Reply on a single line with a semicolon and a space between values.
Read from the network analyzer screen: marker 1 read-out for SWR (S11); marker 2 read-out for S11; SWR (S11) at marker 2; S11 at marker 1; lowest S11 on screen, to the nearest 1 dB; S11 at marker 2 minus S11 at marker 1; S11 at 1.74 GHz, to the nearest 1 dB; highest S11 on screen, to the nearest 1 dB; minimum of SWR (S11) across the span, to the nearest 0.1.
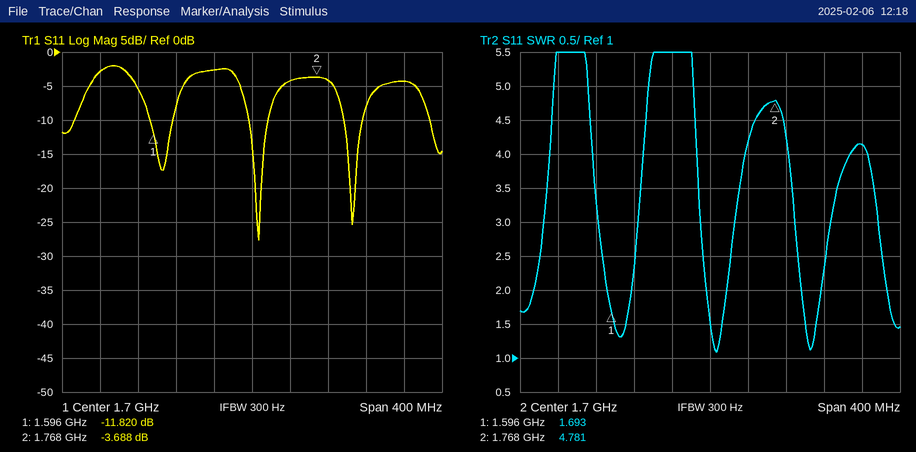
1.693; -3.688 dB; 4.781; -11.820 dB; -28 dB; 8.132 dB; -4 dB; -2 dB; 1.1
